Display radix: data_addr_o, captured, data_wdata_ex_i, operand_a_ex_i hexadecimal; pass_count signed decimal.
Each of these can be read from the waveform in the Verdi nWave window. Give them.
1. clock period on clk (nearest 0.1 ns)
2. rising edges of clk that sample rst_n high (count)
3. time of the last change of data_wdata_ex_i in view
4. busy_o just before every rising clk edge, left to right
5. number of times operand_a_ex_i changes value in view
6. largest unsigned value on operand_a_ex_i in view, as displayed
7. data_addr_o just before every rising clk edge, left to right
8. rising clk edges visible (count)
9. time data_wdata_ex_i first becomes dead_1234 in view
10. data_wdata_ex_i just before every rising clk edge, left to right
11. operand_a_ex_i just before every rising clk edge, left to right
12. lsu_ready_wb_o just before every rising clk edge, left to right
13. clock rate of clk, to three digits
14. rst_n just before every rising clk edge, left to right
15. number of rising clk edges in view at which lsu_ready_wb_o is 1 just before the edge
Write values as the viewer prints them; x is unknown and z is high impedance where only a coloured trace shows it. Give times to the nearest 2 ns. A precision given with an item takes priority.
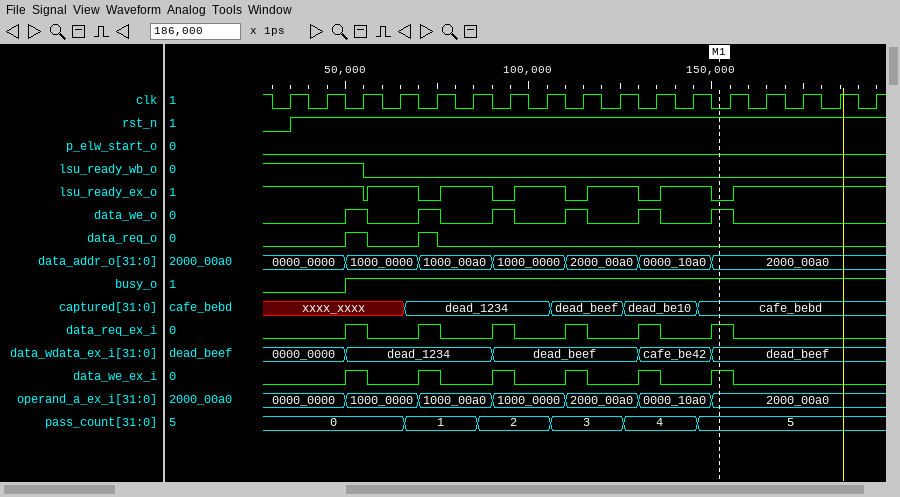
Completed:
10 ns
16
150 ns
0 0 1 1 1 1 1 1 1 1 1 1 1 1 1 1 1
6
2000_00a0
0000_0000, 0000_0000, 1000_0000, 1000_0000, 1000_00a0, 1000_00a0, 1000_0000, 1000_0000, 2000_00a0, 2000_00a0, 0000_10a0, 0000_10a0, 2000_00a0, 2000_00a0, 2000_00a0, 2000_00a0, 2000_00a0
17
50 ns
0000_0000, 0000_0000, dead_1234, dead_1234, dead_1234, dead_1234, dead_beef, dead_beef, dead_beef, dead_beef, cafe_be42, cafe_be42, dead_beef, dead_beef, dead_beef, dead_beef, dead_beef
0000_0000, 0000_0000, 1000_0000, 1000_0000, 1000_00a0, 1000_00a0, 1000_0000, 1000_0000, 2000_00a0, 2000_00a0, 0000_10a0, 0000_10a0, 2000_00a0, 2000_00a0, 2000_00a0, 2000_00a0, 2000_00a0
1 1 1 0 0 0 0 0 0 0 0 0 0 0 0 0 0
100 MHz
0 1 1 1 1 1 1 1 1 1 1 1 1 1 1 1 1
3
